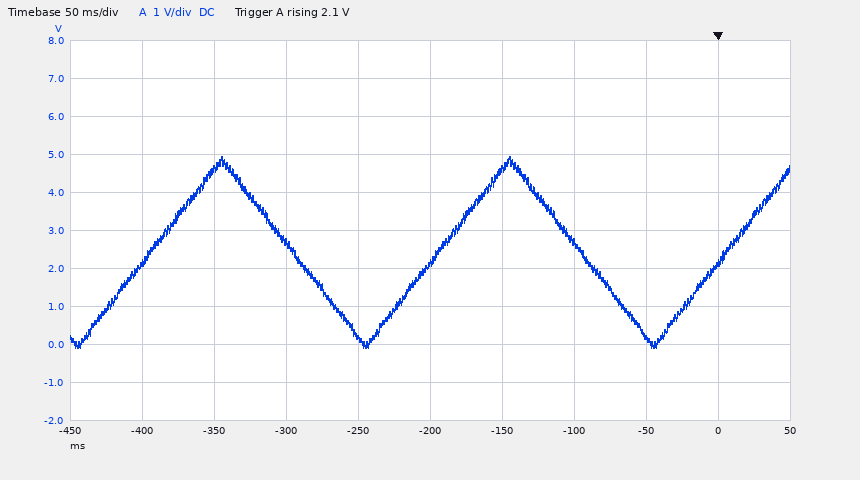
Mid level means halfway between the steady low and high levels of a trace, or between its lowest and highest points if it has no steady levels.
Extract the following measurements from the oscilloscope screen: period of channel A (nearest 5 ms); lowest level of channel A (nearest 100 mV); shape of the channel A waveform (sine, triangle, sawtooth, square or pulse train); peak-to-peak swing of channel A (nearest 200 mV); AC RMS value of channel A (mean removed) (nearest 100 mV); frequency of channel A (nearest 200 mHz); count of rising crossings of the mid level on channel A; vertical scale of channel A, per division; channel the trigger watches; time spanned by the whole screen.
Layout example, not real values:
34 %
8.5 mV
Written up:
200 ms
-100 mV
triangle
5.0 V
1.4 V
5.0 Hz
3
1 V
channel A
500 ms
